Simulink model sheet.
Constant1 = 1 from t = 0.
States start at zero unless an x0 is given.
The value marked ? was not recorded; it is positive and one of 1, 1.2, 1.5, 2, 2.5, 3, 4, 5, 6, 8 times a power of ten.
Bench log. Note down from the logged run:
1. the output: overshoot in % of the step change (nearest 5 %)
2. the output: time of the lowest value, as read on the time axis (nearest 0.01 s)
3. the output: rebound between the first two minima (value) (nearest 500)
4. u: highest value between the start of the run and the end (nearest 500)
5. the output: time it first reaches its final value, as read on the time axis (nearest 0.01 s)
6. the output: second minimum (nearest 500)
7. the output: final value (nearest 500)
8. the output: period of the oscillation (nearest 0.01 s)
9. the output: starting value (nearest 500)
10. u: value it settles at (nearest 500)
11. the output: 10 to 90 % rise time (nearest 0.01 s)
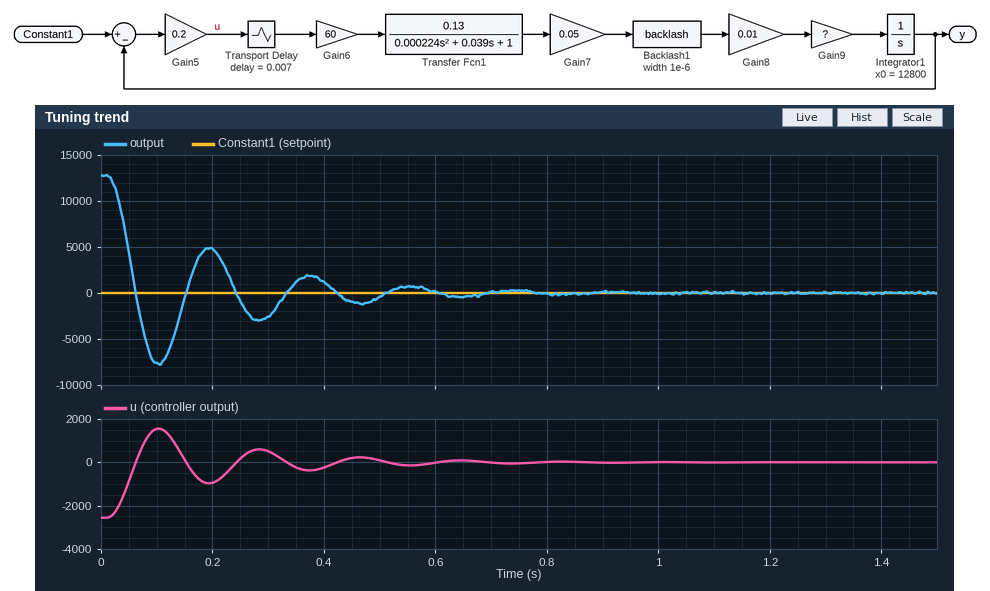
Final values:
60 %
0.10 s
5000
1500
0.06 s
-3000
0
0.18 s
13000
0
0.03 s
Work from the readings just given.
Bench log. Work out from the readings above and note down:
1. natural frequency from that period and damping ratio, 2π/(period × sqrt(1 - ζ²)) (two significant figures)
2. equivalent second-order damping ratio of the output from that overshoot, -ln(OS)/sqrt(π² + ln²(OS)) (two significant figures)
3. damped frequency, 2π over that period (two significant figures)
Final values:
35 rad/s
0.16
35 rad/s
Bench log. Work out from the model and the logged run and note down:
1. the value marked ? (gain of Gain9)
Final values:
60000
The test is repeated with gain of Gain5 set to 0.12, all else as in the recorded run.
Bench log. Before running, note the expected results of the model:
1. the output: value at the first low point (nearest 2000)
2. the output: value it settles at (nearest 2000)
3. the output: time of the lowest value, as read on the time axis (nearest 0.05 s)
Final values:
-4000
0
0.15 s
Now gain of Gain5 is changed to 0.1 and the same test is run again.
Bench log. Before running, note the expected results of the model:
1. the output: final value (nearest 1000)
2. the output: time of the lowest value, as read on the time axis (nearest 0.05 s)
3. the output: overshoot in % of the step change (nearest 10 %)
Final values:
0
0.15 s
30 %
